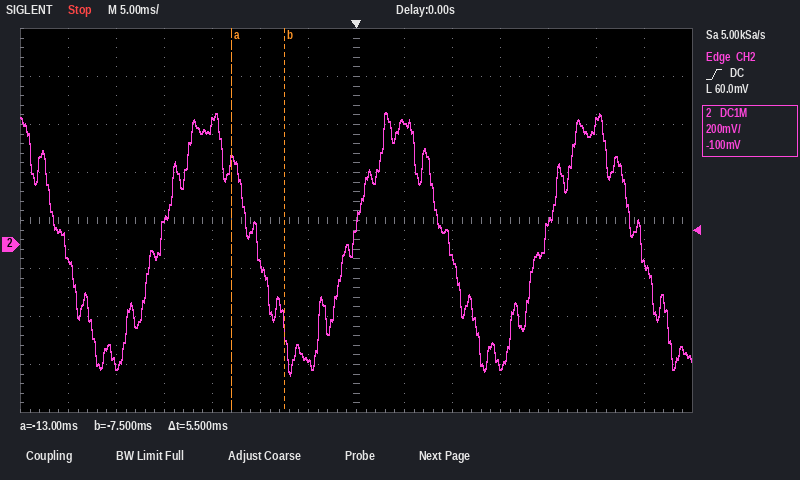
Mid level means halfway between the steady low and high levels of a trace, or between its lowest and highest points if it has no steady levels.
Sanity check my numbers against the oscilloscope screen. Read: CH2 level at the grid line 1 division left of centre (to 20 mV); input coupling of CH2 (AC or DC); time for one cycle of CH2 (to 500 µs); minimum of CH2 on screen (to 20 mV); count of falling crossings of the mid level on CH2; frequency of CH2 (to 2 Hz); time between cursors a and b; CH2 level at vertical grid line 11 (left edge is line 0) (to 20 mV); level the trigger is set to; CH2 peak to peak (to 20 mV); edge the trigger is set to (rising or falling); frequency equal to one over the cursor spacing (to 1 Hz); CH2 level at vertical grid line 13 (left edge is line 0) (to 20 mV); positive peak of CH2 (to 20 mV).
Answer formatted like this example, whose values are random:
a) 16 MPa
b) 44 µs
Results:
a) -480 mV
b) DC
c) 20.0 ms
d) -540 mV
e) 4
f) 50 Hz
g) 5.5 ms
h) 100 mV
i) 60.0 mV
j) 1.10 V
k) rising
l) 182 Hz
m) -80 mV
n) 560 mV
